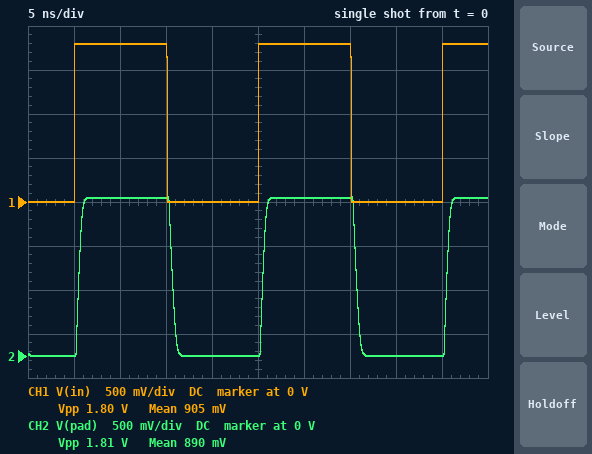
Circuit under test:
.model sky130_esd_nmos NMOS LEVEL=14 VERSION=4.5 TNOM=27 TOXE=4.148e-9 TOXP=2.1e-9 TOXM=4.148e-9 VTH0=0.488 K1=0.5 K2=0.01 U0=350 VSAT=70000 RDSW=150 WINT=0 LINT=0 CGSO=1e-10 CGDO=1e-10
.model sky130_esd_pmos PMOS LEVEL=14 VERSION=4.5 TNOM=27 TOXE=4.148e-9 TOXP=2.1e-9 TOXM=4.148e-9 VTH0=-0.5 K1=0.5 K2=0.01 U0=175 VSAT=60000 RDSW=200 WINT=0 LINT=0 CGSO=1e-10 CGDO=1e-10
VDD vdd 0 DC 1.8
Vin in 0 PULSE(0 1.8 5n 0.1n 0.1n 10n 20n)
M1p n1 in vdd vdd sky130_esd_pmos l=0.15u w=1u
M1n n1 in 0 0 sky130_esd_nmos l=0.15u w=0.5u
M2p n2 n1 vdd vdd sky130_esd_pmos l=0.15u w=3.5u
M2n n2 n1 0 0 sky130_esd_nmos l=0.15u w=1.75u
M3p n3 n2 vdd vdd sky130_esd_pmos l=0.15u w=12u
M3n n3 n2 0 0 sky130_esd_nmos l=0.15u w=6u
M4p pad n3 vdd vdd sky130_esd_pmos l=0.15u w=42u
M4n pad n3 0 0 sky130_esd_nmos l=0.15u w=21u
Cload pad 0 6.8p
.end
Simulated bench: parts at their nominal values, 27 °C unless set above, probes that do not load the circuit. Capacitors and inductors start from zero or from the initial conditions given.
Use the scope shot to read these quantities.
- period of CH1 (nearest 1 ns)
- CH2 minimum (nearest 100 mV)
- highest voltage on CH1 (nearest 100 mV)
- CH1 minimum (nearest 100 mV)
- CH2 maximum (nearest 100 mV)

20 ns
0 V
1.8 V
0 V
1.8 V
